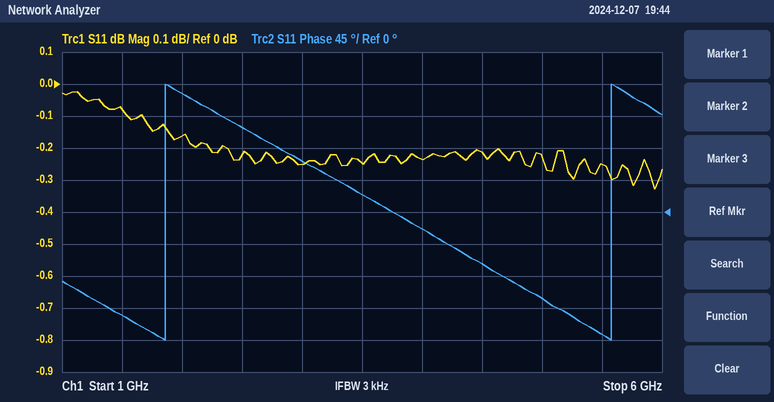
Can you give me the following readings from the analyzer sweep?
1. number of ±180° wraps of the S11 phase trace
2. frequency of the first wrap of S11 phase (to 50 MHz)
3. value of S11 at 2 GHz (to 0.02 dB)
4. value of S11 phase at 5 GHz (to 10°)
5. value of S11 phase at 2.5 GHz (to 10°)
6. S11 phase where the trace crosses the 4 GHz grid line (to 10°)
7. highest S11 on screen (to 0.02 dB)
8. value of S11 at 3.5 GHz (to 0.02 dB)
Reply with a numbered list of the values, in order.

1. 2
2. 1.85 GHz
3. -0.16 dB
4. -120°
5. 120°
6. -20°
7. -0.02 dB
8. -0.24 dB
